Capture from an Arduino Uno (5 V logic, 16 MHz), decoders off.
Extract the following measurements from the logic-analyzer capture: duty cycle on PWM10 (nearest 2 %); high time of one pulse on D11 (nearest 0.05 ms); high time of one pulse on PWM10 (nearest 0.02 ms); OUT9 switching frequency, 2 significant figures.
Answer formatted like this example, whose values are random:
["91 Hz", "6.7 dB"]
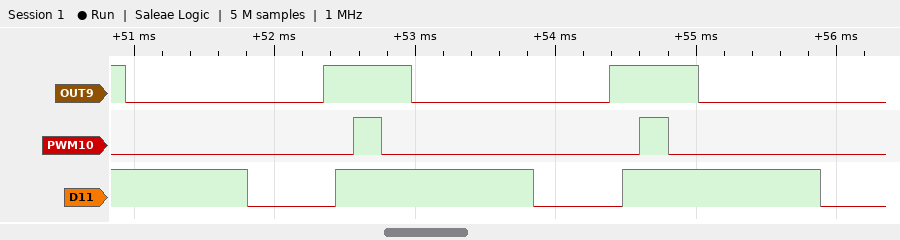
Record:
["10 %", "1.40 ms", "0.20 ms", "490 Hz"]
